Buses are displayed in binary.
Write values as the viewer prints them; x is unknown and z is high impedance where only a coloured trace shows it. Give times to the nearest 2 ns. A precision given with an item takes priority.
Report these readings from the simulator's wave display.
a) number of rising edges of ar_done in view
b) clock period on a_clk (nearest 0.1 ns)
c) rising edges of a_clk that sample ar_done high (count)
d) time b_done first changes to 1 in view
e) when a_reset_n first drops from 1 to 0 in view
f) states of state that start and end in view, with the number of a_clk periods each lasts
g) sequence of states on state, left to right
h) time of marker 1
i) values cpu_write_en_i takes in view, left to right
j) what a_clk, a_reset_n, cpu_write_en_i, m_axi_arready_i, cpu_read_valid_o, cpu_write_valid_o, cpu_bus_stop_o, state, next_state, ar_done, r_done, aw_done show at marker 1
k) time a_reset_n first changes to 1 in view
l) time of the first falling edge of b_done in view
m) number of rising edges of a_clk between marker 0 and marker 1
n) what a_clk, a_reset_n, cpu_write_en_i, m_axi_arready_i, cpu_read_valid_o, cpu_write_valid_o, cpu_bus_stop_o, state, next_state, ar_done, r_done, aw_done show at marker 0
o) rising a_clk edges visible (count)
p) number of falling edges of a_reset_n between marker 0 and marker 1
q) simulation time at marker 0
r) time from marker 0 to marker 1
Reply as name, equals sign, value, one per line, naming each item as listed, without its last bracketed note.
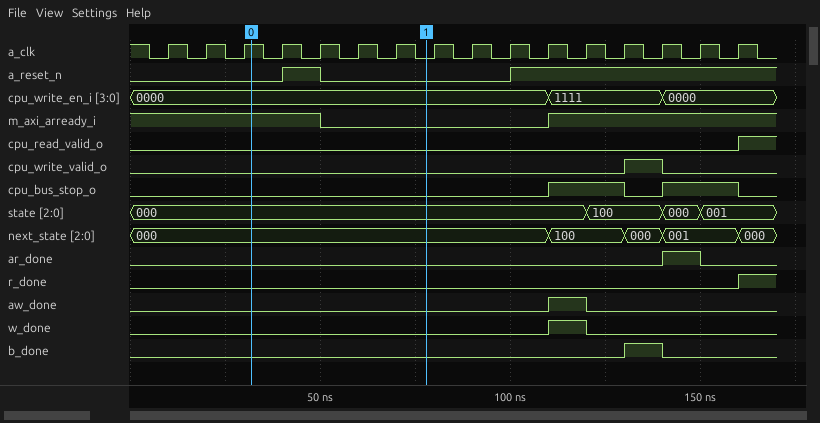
number of rising edges of ar_done in view = 1
clock period on a_clk = 10 ns
rising edges of a_clk that sample ar_done high = 1
time b_done first changes to 1 in view = 130 ns
when a_reset_n first drops from 1 to 0 in view = 50 ns
states of state that start and end in view, with the number of a_clk periods each lasts = 100: 2, 000: 1
sequence of states on state, left to right = 000, 100, 000, 001
time of marker 1 = 78 ns
values cpu_write_en_i takes in view, left to right = 0000, 1111, 0000
what a_clk, a_reset_n, cpu_write_en_i, m_axi_arready_i, cpu_read_valid_o, cpu_write_valid_o, cpu_bus_stop_o, state, next_state, ar_done, r_done, aw_done show at marker 1 = a_clk=0, a_reset_n=0, cpu_write_en_i=0000, m_axi_arready_i=0, cpu_read_valid_o=0, cpu_write_valid_o=0, cpu_bus_stop_o=0, state=000, next_state=000, ar_done=0, r_done=0, aw_done=0
time a_reset_n first changes to 1 in view = 40 ns
time of the first falling edge of b_done in view = 140 ns
number of rising edges of a_clk between marker 0 and marker 1 = 4
what a_clk, a_reset_n, cpu_write_en_i, m_axi_arready_i, cpu_read_valid_o, cpu_write_valid_o, cpu_bus_stop_o, state, next_state, ar_done, r_done, aw_done show at marker 0 = a_clk=1, a_reset_n=0, cpu_write_en_i=0000, m_axi_arready_i=1, cpu_read_valid_o=0, cpu_write_valid_o=0, cpu_bus_stop_o=0, state=000, next_state=000, ar_done=0, r_done=0, aw_done=0
rising a_clk edges visible = 16
number of falling edges of a_reset_n between marker 0 and marker 1 = 1
simulation time at marker 0 = 32 ns
time from marker 0 to marker 1 = 46 ns
